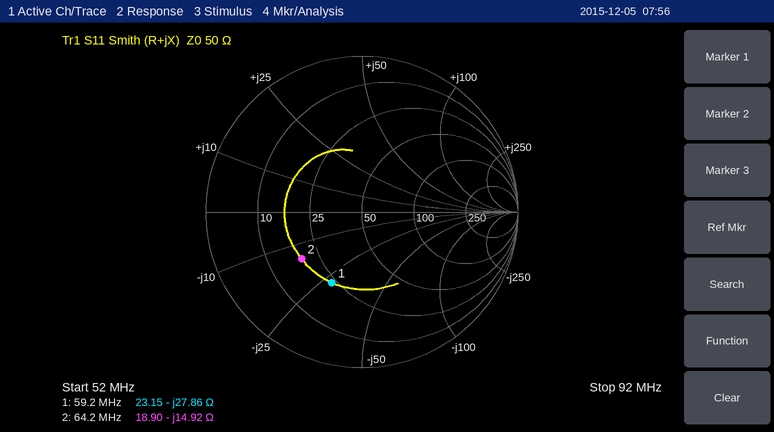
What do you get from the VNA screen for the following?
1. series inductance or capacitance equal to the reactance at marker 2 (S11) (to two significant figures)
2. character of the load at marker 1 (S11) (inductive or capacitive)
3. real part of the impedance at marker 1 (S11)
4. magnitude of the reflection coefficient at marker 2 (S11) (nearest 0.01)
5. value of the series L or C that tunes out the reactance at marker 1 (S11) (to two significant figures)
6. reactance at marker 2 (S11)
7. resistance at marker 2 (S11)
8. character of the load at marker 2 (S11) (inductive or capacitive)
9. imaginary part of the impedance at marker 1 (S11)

170 pF
capacitive
23.15 Ω
0.49
75 nH
-14.92 Ω
18.90 Ω
capacitive
-27.86 Ω
